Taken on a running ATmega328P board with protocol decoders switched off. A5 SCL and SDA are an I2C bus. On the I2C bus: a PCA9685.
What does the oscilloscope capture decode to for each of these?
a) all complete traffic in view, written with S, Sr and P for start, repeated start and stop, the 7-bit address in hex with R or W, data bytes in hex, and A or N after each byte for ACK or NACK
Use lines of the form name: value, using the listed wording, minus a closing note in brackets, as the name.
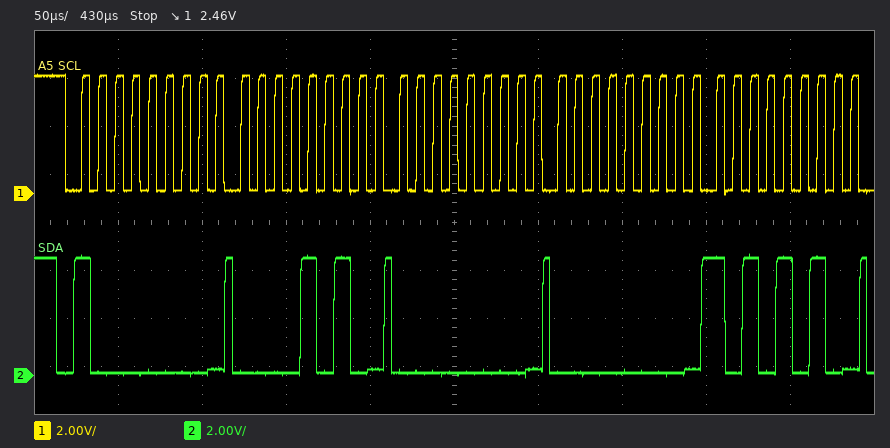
all complete traffic in view, written with S, Sr and P for start, repeated start and stop, the 7-bit address in hex with R or W, data bytes in hex, and A or N after each byte for ACK or NACK: S 40W A 0A A 00 A 00 A AA A
